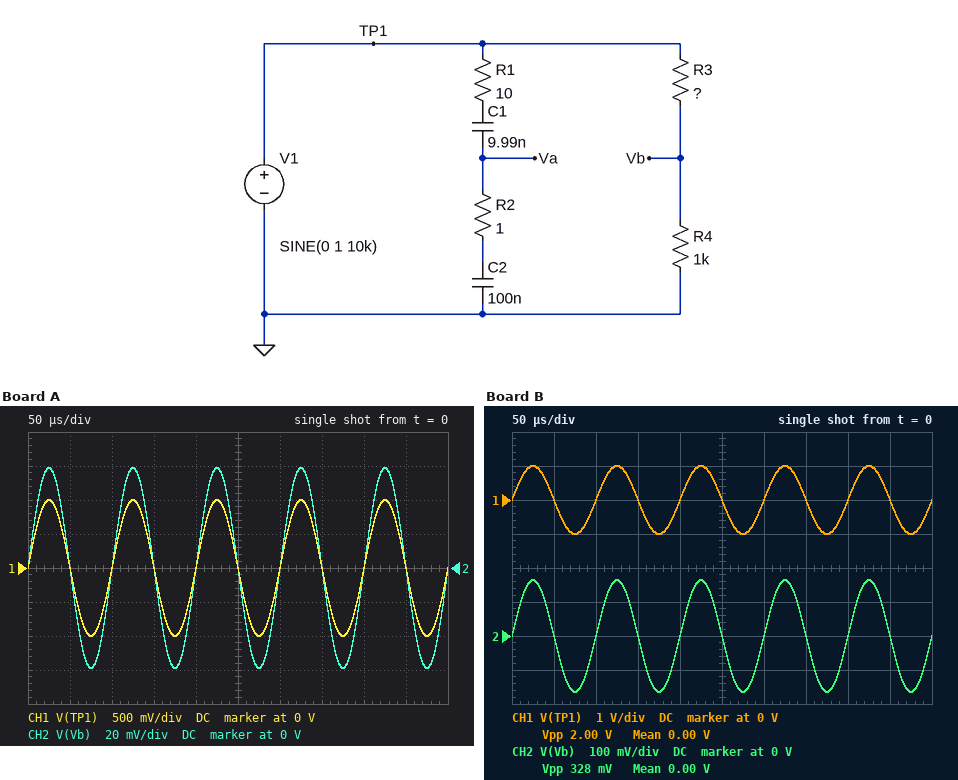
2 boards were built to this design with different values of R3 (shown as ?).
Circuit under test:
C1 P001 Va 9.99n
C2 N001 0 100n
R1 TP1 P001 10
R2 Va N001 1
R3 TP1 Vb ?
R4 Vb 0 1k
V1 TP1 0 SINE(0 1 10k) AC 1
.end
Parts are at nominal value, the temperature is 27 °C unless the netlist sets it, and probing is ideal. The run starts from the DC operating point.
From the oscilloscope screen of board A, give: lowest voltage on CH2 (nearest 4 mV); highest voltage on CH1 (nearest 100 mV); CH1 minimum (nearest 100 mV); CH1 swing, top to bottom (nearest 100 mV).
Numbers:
-60 mV
1.0 V
-1.0 V
2.0 V
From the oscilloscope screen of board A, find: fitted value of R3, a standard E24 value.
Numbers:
16 kΩ
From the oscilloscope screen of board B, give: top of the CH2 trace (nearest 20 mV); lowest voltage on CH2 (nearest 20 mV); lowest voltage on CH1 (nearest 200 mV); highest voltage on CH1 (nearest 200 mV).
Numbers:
160 mV
-160 mV
-1.0 V
1.0 V
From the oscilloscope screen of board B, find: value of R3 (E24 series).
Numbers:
5.1 kΩ
